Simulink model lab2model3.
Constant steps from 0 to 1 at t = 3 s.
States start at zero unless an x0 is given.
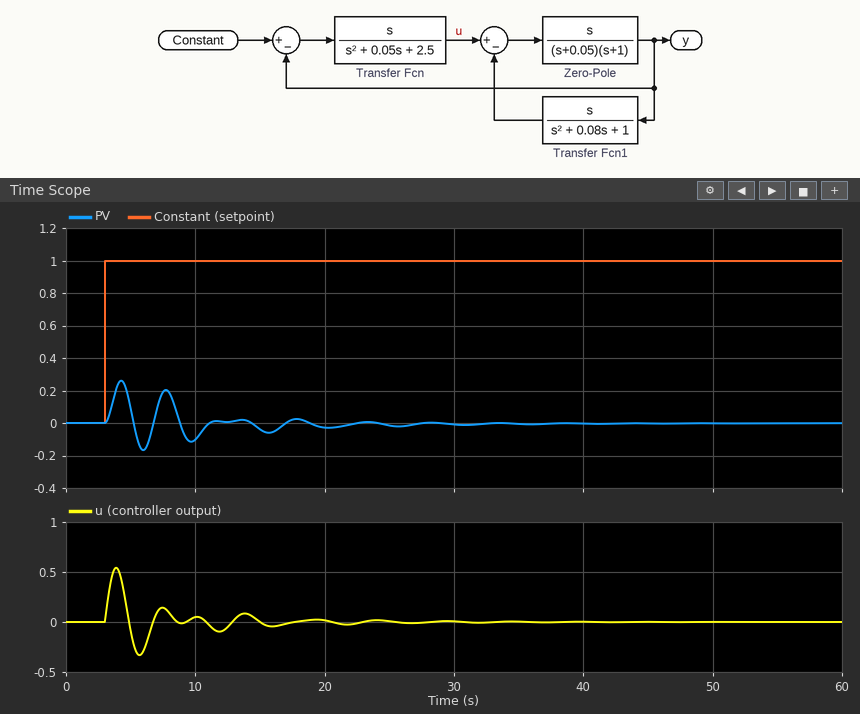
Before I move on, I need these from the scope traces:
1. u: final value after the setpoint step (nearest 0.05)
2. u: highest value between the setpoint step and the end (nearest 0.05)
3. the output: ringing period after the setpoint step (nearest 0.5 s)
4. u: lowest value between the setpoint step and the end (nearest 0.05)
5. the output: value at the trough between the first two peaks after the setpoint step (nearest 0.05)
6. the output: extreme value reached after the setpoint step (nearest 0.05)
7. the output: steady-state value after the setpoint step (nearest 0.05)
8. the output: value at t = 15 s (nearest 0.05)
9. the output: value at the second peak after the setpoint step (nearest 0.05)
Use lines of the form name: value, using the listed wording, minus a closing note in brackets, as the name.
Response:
u: final value after the setpoint step: 0.00
u: highest value between the setpoint step and the end: 0.55
the output: ringing period after the setpoint step: 3.5 s
u: lowest value between the setpoint step and the end: -0.35
the output: value at the trough between the first two peaks after the setpoint step: -0.15
the output: extreme value reached after the setpoint step: 0.25
the output: steady-state value after the setpoint step: 0.00
the output: value at t = 15 s: -0.05
the output: value at the second peak after the setpoint step: 0.20
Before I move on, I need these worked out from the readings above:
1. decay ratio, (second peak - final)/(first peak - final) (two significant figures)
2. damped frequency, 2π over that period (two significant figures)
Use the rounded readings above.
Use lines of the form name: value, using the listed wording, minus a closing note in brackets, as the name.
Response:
decay ratio, (second peak - final)/(first peak - final): 0.80
damped frequency, 2π over that period: 1.8 rad/s
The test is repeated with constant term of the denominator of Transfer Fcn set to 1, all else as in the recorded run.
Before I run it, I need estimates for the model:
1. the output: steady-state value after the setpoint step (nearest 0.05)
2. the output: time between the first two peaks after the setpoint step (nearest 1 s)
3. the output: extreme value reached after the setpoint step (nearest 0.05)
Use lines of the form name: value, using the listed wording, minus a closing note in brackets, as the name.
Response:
the output: steady-state value after the setpoint step: 0.00
the output: time between the first two peaks after the setpoint step: 4 s
the output: extreme value reached after the setpoint step: 0.40
